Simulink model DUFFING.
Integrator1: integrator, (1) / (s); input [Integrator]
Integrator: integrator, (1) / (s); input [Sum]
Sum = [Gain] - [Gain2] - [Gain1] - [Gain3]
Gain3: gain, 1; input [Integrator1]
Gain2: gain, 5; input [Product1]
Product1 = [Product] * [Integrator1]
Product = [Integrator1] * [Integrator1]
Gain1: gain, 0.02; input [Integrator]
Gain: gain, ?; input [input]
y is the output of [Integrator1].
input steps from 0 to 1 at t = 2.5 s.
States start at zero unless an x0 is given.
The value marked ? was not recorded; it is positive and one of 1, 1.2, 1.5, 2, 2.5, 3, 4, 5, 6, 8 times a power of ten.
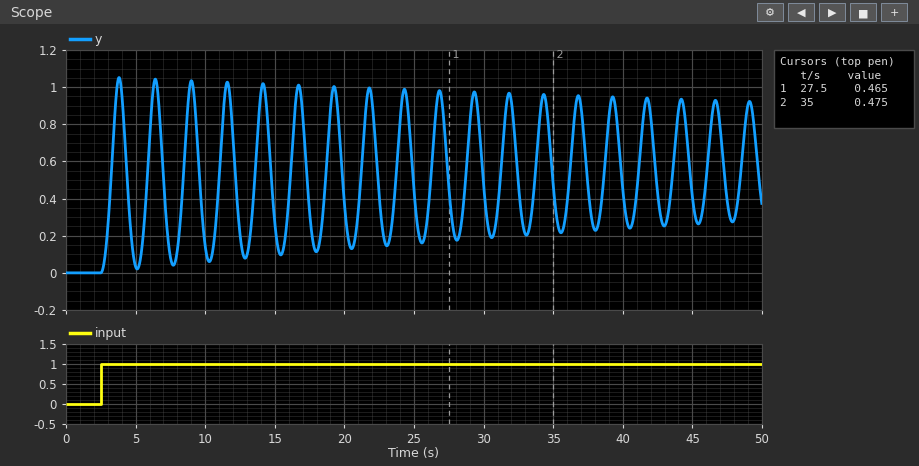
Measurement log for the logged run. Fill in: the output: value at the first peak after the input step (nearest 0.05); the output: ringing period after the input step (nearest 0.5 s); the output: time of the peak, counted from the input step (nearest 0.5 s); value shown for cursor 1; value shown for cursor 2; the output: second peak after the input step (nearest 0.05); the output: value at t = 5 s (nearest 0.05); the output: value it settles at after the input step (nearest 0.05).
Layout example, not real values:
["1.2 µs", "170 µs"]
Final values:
["1.05", "2.5 s", "1.5 s", "0.465", "0.475", "1.05", "0.05", "0.65"]
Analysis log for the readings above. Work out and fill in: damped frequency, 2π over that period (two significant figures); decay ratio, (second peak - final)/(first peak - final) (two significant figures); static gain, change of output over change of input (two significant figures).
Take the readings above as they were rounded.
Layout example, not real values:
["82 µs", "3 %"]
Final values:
["2.5 rad/s", "1.0", "0.65"]
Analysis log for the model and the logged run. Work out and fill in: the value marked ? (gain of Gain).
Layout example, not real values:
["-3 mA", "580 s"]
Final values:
["2"]
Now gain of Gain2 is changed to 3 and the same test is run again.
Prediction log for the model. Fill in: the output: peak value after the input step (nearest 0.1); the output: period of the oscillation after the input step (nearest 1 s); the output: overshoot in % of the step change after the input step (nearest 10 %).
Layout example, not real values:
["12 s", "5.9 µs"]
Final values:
["1.2", "3 s", "70 %"]
